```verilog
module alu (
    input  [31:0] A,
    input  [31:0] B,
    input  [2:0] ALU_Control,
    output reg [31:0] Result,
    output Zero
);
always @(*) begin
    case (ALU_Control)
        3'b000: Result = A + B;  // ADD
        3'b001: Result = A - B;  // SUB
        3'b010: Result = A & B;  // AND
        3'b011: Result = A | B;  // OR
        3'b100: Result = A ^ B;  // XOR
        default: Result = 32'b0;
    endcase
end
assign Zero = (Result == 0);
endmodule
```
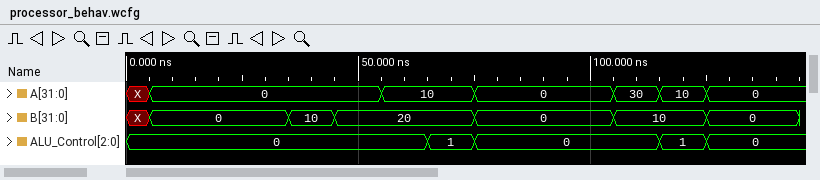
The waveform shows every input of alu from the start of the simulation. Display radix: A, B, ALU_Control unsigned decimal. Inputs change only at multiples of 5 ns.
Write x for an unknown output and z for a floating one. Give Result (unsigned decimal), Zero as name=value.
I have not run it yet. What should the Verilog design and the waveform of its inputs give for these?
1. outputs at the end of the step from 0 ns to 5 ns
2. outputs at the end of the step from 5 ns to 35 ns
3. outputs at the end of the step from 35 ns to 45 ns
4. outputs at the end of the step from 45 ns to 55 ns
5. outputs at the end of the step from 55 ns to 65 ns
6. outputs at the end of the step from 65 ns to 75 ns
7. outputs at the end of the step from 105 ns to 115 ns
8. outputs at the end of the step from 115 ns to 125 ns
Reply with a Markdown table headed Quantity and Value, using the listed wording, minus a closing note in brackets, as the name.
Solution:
| Quantity | Value |
|---|---|
| outputs at the end of the step from 0 ns to 5 ns | Result=x, Zero=x |
| outputs at the end of the step from 5 ns to 35 ns | Result=0, Zero=1 |
| outputs at the end of the step from 35 ns to 45 ns | Result=10, Zero=0 |
| outputs at the end of the step from 45 ns to 55 ns | Result=20, Zero=0 |
| outputs at the end of the step from 55 ns to 65 ns | Result=30, Zero=0 |
| outputs at the end of the step from 65 ns to 75 ns | Result=4294967286, Zero=0 |
| outputs at the end of the step from 105 ns to 115 ns | Result=40, Zero=0 |
| outputs at the end of the step from 115 ns to 125 ns | Result=0, Zero=1 |
